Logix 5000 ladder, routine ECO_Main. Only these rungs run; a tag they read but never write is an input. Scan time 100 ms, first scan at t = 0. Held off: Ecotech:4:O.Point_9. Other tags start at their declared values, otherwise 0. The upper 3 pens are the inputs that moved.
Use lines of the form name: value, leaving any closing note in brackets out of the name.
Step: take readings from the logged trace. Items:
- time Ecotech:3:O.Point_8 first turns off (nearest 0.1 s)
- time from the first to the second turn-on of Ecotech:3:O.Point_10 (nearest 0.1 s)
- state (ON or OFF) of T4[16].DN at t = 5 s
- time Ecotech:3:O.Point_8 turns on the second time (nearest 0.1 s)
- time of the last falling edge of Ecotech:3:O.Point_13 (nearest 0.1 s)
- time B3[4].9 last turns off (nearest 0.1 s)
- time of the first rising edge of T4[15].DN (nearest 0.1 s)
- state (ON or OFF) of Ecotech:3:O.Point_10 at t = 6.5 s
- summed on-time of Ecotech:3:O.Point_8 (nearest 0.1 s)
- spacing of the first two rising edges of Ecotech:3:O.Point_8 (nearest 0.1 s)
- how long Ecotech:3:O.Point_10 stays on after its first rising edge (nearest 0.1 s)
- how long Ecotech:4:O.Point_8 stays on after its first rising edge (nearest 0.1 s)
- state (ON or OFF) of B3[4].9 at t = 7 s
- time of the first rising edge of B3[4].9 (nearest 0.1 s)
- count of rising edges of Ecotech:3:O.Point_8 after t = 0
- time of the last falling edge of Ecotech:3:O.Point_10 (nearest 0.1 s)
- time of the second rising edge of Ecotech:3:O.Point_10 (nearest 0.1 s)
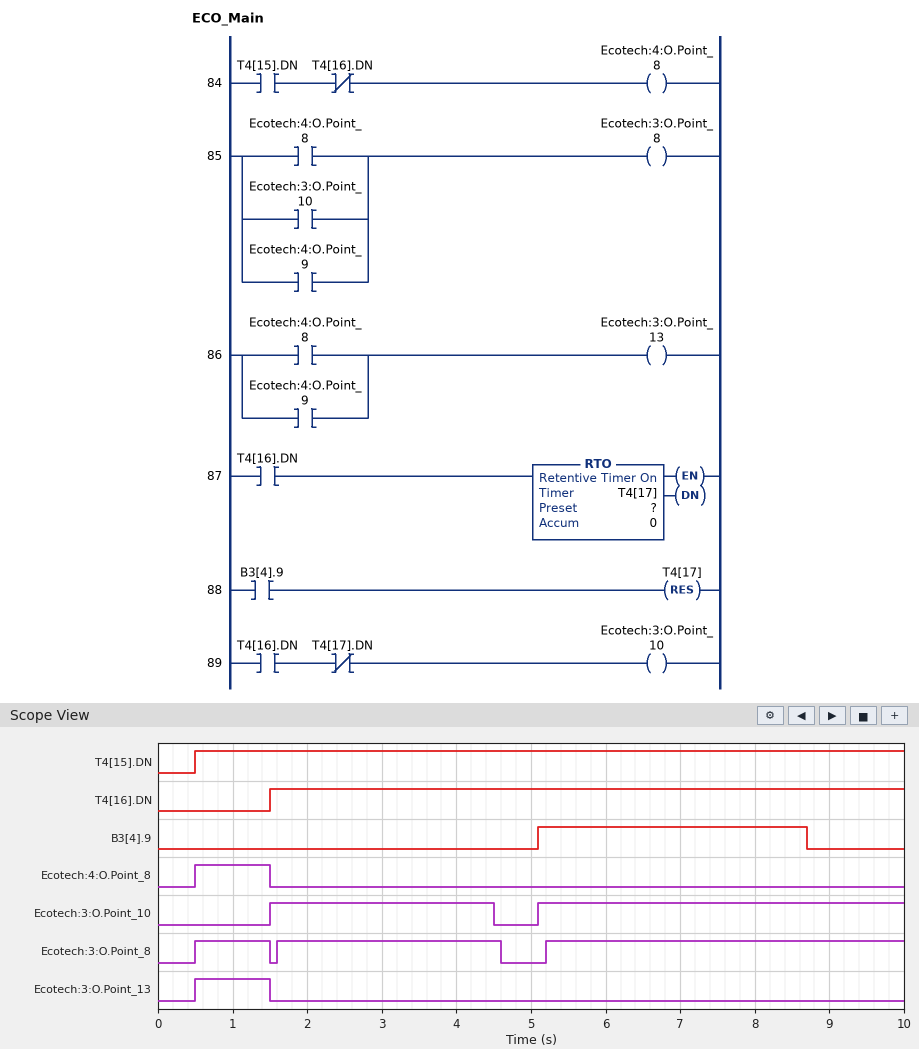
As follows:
time Ecotech:3:O.Point_8 first turns off: 1.5 s
time from the first to the second turn-on of Ecotech:3:O.Point_10: 3.6 s
state (ON or OFF) of T4[16].DN at t = 5 s: ON
time Ecotech:3:O.Point_8 turns on the second time: 1.6 s
time of the last falling edge of Ecotech:3:O.Point_13: 1.5 s
time B3[4].9 last turns off: 8.7 s
time of the first rising edge of T4[15].DN: 0.5 s
state (ON or OFF) of Ecotech:3:O.Point_10 at t = 6.5 s: ON
summed on-time of Ecotech:3:O.Point_8: 8.8 s
spacing of the first two rising edges of Ecotech:3:O.Point_8: 1.1 s
how long Ecotech:3:O.Point_10 stays on after its first rising edge: 3.0 s
how long Ecotech:4:O.Point_8 stays on after its first rising edge: 1.0 s
state (ON or OFF) of B3[4].9 at t = 7 s: ON
time of the first rising edge of B3[4].9: 5.1 s
count of rising edges of Ecotech:3:O.Point_8 after t = 0: 3
time of the last falling edge of Ecotech:3:O.Point_10: 4.5 s
time of the second rising edge of Ecotech:3:O.Point_10: 5.1 s
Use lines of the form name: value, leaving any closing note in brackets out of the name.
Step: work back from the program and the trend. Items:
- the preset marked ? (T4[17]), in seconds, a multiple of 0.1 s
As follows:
the preset marked ? (T4[17]), in seconds, a multiple of 0.1 s: 3.0 s
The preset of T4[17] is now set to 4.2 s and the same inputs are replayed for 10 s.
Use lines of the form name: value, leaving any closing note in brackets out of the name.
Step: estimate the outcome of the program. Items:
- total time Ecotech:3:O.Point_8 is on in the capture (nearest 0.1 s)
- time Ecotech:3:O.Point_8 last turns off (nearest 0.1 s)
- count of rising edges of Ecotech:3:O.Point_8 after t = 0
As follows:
total time Ecotech:3:O.Point_8 is on in the capture: 9.4 s
time Ecotech:3:O.Point_8 last turns off: 1.5 s
count of rising edges of Ecotech:3:O.Point_8 after t = 0: 2
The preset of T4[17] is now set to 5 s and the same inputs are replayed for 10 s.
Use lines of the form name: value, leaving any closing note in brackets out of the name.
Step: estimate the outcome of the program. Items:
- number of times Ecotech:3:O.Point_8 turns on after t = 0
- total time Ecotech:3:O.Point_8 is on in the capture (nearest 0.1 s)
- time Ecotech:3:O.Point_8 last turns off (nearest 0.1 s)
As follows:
number of times Ecotech:3:O.Point_8 turns on after t = 0: 2
total time Ecotech:3:O.Point_8 is on in the capture: 9.4 s
time Ecotech:3:O.Point_8 last turns off: 1.5 s
